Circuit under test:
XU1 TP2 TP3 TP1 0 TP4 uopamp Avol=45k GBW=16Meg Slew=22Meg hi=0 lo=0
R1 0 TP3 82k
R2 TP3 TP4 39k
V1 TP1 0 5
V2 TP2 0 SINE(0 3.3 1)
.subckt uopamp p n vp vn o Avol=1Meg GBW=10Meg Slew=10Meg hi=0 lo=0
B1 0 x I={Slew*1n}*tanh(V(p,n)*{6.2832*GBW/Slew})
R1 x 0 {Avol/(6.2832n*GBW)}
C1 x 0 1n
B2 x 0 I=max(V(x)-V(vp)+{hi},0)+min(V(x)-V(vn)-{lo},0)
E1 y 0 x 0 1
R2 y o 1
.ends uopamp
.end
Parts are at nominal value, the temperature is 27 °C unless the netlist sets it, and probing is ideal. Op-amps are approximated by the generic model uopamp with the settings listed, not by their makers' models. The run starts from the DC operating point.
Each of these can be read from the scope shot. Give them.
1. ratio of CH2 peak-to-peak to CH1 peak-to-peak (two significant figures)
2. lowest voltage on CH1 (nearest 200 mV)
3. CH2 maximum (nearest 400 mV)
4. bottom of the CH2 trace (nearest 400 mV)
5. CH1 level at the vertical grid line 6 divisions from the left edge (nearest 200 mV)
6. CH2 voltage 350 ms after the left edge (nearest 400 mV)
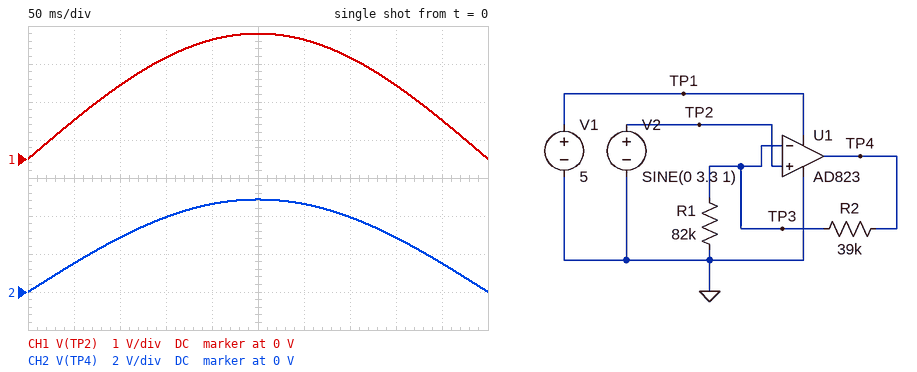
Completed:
1.5
0 V
4.8 V
0 V
3.2 V
4.0 V
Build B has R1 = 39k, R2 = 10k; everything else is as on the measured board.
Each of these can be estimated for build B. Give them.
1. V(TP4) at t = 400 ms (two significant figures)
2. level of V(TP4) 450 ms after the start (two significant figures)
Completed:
2.4 V
1.3 V
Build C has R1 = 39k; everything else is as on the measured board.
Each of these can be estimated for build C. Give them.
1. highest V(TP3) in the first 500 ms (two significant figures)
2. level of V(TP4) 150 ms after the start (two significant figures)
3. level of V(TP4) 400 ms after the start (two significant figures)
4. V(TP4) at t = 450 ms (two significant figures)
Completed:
2.5 V
5.0 V
3.9 V
2.0 V
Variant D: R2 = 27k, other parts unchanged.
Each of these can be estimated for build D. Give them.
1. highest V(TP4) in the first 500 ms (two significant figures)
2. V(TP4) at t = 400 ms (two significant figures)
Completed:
4.4 V
2.6 V
